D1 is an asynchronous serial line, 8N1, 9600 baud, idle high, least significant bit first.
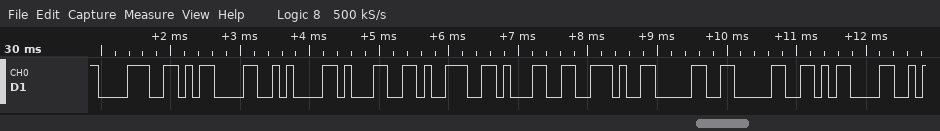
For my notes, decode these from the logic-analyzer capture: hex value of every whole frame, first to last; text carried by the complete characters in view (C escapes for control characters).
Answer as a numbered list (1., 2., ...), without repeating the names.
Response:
1. 0x38 0x0D 0x0A 0x31 0x39 0x31 0x2E 0x30 0x30 0x0D
2. "8\r\n191.00\r"
